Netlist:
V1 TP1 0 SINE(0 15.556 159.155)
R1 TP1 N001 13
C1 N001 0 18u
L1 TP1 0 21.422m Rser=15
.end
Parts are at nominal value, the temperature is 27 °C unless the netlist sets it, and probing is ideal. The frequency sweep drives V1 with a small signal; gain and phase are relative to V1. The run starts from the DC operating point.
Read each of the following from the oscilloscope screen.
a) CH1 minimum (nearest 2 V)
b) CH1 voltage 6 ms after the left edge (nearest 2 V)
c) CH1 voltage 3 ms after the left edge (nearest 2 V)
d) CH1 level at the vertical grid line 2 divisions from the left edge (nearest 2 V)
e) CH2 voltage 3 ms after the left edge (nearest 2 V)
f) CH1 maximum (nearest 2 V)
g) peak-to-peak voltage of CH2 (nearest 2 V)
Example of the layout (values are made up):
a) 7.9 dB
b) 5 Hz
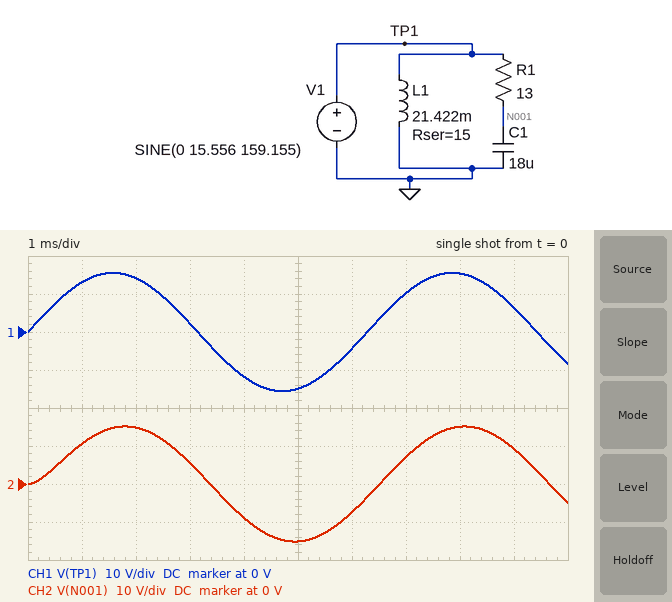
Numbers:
a) -16 V
b) -4 V
c) 2 V
d) 14 V
e) 6 V
f) 16 V
g) 30 V
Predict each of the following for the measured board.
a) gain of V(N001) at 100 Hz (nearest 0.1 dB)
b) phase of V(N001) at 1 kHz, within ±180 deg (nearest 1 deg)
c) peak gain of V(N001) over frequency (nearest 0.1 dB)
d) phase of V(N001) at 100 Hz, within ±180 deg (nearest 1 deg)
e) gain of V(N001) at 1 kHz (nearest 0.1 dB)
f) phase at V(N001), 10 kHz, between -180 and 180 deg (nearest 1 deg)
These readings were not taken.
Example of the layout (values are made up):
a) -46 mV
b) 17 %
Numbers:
a) -0.1 dB
b) -56 deg
c) 0 dB
d) -8 deg
e) -5.0 dB
f) -86 deg
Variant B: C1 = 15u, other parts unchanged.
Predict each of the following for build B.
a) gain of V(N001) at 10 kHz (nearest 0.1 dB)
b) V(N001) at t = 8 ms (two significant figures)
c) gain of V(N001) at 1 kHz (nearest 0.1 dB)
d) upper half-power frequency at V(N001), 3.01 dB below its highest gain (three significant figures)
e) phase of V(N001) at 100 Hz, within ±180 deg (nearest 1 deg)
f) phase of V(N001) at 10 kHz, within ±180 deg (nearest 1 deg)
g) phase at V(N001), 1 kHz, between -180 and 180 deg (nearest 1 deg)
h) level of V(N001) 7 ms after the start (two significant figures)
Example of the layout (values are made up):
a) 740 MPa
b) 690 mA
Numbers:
a) -21.8 dB
b) 15 V
c) -4.0 dB
d) 816 Hz
e) -7 deg
f) -85 deg
g) -51 deg
h) 7.6 V
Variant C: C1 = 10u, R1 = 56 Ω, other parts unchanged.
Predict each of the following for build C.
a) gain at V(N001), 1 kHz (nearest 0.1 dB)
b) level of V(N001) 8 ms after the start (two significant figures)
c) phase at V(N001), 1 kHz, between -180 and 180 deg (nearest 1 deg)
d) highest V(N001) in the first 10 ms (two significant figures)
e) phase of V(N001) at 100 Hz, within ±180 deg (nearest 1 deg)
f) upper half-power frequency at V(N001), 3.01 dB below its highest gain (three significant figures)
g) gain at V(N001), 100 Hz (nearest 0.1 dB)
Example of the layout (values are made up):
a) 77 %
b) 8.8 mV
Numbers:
a) -11.3 dB
b) 13 V
c) -74 deg
d) 14 V
e) -19 deg
f) 284 Hz
g) -0.5 dB
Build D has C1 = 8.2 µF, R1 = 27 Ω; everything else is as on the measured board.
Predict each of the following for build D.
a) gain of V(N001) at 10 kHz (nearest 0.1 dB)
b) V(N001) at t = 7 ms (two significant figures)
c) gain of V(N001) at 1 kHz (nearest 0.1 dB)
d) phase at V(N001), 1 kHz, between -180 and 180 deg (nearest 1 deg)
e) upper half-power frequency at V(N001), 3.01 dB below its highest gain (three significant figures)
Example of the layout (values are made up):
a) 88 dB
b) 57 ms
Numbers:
a) -22.9 dB
b) 7.3 V
c) -4.7 dB
d) -54 deg
e) 719 Hz
